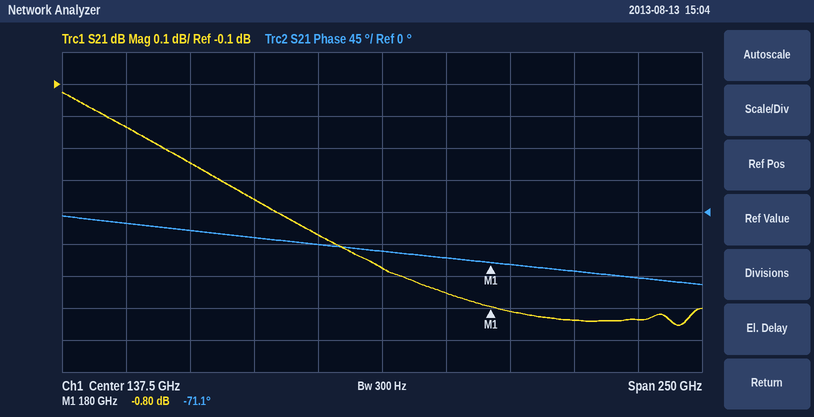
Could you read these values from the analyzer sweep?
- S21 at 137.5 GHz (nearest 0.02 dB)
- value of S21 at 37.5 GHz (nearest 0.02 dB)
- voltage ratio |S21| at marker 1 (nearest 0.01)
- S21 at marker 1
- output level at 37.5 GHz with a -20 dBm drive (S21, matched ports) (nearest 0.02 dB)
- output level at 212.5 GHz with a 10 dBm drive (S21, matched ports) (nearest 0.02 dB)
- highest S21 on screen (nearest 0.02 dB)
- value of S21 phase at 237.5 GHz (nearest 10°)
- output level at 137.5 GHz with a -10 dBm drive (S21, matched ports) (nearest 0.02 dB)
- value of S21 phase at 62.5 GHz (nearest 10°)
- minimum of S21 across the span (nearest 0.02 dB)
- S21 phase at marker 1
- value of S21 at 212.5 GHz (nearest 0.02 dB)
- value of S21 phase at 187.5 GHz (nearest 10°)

-0.68 dB
-0.24 dB
0.91
-0.80 dB
-20.24 dBm
9.16 dBm
-0.12 dB
-90°
-10.68 dBm
-30°
-0.86 dB
-71.1°
-0.84 dB
-70°
